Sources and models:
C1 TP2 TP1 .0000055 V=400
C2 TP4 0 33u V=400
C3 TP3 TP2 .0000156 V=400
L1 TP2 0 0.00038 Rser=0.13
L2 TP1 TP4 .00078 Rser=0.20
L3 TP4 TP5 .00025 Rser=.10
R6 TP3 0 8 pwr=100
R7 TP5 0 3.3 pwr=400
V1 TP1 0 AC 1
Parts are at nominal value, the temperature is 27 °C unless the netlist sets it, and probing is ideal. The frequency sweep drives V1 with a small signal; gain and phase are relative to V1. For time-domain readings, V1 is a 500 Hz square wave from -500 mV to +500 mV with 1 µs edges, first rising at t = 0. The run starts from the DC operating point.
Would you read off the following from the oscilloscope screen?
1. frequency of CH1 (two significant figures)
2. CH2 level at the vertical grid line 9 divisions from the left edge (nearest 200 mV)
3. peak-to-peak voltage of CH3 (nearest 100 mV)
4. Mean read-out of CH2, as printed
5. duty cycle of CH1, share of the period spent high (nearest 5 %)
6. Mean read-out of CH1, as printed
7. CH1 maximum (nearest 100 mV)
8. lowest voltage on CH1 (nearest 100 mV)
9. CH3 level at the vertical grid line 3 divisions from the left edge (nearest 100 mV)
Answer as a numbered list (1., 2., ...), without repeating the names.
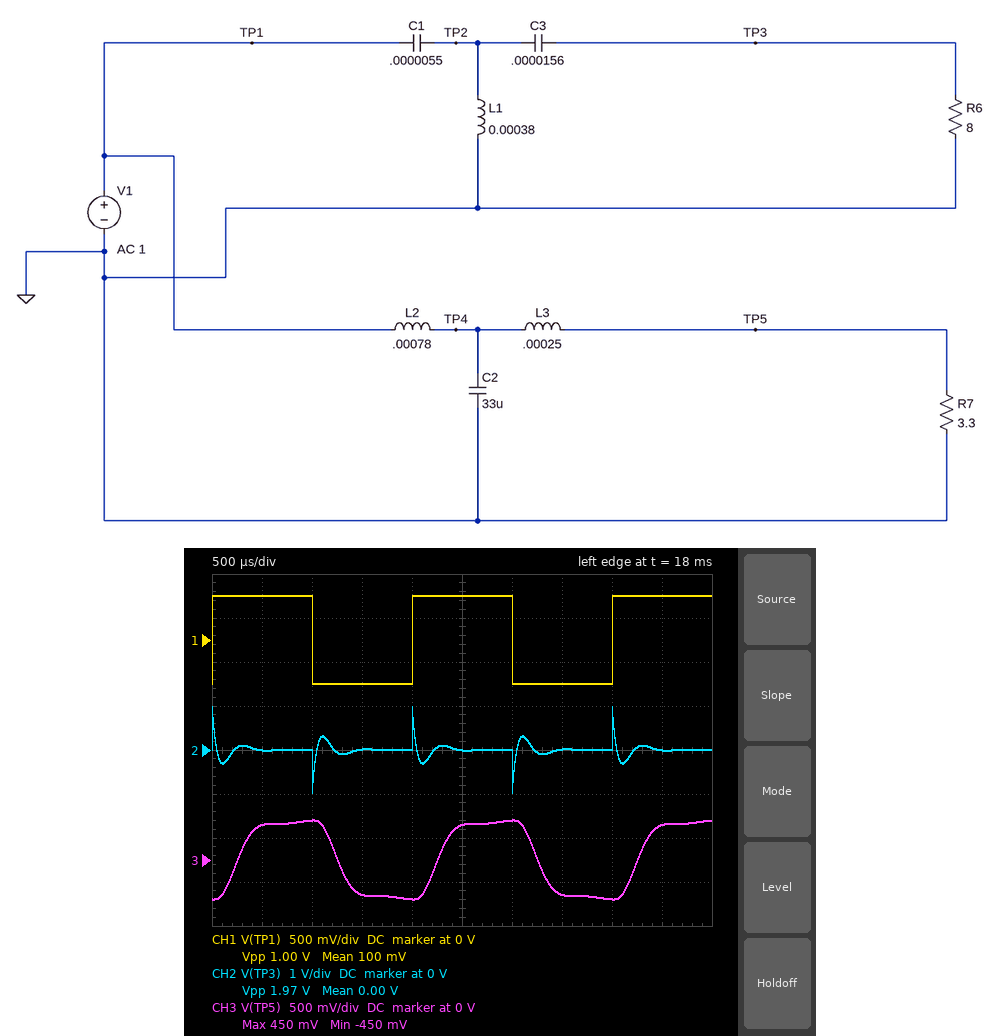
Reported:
1. 500 Hz
2. 0 V
3. 900 mV
4. 0.00 V
5. 50 %
6. 100 mV
7. 500 mV
8. -500 mV
9. -400 mV
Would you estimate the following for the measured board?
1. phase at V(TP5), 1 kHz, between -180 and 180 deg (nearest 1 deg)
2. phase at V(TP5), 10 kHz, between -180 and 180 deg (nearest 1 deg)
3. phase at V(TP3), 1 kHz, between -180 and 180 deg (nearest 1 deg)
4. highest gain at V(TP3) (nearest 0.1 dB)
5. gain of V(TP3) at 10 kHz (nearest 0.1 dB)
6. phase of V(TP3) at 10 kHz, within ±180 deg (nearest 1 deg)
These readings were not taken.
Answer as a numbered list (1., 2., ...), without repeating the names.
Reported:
1. -89 deg
2. 103 deg
3. -140 deg
4. 0 dB
5. 0 dB
6. 28 deg
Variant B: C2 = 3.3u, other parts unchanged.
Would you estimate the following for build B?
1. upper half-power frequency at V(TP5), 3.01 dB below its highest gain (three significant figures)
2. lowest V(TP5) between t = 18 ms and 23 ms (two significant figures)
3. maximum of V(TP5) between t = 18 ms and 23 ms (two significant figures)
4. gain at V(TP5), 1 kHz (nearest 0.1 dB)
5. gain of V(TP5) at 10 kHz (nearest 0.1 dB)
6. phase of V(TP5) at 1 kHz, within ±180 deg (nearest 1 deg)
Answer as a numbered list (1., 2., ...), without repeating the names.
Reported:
1. 577 Hz
2. -430 mV
3. 430 mV
4. -6.7 dB
5. -29.6 dB
6. -63 deg
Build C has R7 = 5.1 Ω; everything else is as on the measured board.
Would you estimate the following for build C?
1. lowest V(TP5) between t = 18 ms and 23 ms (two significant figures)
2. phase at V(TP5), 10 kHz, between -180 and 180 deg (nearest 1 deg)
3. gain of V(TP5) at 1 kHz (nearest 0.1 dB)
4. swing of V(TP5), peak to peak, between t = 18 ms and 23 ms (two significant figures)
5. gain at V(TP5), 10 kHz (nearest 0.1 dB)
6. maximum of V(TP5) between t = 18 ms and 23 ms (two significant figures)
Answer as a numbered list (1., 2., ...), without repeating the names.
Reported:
1. -600 mV
2. 109 deg
3. 0 dB
4. 1.2 V
5. -50.0 dB
6. 600 mV
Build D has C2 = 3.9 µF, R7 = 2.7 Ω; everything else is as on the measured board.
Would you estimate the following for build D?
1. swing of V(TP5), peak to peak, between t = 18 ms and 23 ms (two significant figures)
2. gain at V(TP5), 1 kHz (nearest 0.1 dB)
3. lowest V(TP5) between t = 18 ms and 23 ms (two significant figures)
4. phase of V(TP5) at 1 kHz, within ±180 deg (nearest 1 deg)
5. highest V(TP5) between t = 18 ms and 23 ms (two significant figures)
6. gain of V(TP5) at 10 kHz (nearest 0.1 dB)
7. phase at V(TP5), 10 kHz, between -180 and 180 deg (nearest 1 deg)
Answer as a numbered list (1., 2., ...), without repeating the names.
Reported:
1. 810 mV
2. -8.1 dB
3. -410 mV
4. -67 deg
5. 410 mV
6. -33.5 dB
7. 104 deg
